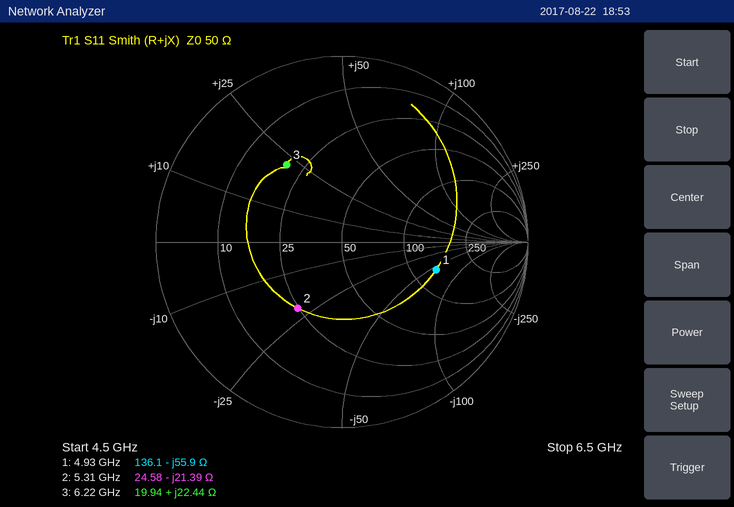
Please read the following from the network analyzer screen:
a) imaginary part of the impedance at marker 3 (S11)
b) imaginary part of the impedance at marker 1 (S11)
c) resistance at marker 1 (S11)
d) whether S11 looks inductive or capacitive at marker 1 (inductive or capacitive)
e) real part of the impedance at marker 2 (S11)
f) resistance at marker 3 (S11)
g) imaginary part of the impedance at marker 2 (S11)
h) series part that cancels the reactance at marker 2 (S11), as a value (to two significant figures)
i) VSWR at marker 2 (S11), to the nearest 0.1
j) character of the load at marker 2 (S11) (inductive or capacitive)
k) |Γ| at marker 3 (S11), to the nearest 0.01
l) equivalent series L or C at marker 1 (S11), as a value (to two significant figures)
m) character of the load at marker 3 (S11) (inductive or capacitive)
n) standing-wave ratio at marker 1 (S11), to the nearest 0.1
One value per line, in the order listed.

+22.44 Ω
-55.9 Ω
136.1 Ω
capacitive
24.58 Ω
19.94 Ω
-21.39 Ω
640 pH
2.5
capacitive
0.51
580 fF
inductive
3.2
